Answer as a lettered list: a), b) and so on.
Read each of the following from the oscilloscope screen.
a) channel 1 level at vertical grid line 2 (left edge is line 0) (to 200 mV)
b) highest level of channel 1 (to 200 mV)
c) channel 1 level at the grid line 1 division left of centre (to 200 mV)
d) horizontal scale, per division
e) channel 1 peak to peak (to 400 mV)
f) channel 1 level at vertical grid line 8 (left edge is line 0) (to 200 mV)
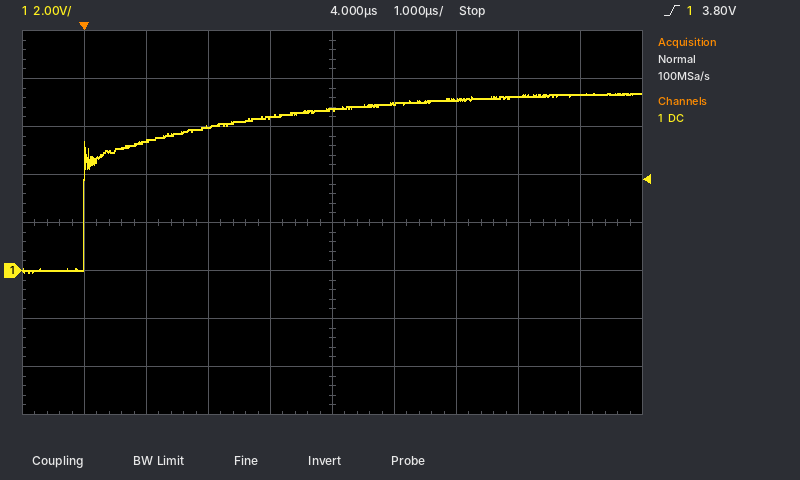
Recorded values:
a) 5.4 V
b) 7.4 V
c) 6.4 V
d) 1 µs
e) 7.6 V
f) 7.2 V
